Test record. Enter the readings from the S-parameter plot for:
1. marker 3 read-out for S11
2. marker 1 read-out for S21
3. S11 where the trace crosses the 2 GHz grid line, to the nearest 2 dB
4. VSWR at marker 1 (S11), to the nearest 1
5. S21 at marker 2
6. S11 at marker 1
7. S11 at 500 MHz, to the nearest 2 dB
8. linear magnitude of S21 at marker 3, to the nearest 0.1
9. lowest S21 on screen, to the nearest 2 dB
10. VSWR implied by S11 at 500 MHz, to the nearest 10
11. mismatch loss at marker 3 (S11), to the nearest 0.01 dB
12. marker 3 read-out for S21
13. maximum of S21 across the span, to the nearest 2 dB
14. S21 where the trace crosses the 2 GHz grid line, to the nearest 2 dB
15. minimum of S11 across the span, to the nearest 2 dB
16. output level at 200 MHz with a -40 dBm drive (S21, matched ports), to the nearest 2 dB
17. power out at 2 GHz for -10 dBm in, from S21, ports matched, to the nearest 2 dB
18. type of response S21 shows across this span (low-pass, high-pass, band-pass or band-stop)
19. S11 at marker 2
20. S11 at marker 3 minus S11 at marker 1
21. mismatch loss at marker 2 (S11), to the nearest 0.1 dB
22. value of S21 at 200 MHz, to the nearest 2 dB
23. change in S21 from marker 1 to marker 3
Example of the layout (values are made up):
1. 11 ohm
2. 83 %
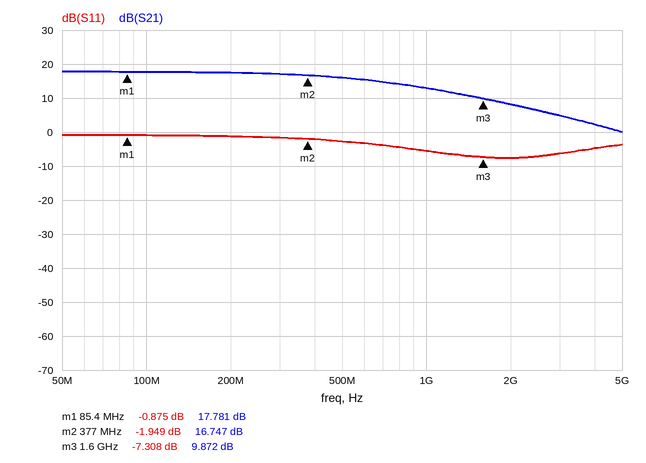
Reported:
1. -7.308 dB
2. 17.781 dB
3. -8 dB
4. 20
5. 16.747 dB
6. -0.875 dB
7. -2 dB
8. 3.1
9. 0 dB
10. 10
11. 0.89 dB
12. 9.872 dB
13. 18 dB
14. 8 dB
15. -8 dB
16. -22 dBm
17. -2 dBm
18. low-pass
19. -1.949 dB
20. -6.433 dB
21. 4.4 dB
22. 18 dB
23. -7.909 dB
